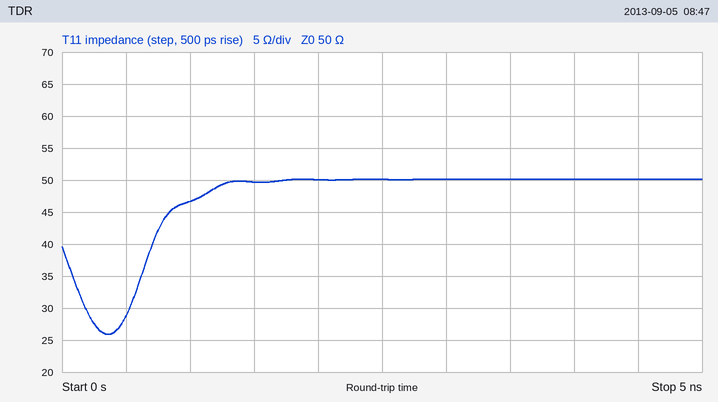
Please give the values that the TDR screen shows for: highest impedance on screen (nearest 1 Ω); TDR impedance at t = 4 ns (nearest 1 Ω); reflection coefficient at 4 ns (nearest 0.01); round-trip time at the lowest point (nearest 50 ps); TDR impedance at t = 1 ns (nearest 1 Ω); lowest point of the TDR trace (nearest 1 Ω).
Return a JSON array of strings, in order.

["50 Ω", "50 Ω", "0.00", "350 ps", "47 Ω", "26 Ω"]
